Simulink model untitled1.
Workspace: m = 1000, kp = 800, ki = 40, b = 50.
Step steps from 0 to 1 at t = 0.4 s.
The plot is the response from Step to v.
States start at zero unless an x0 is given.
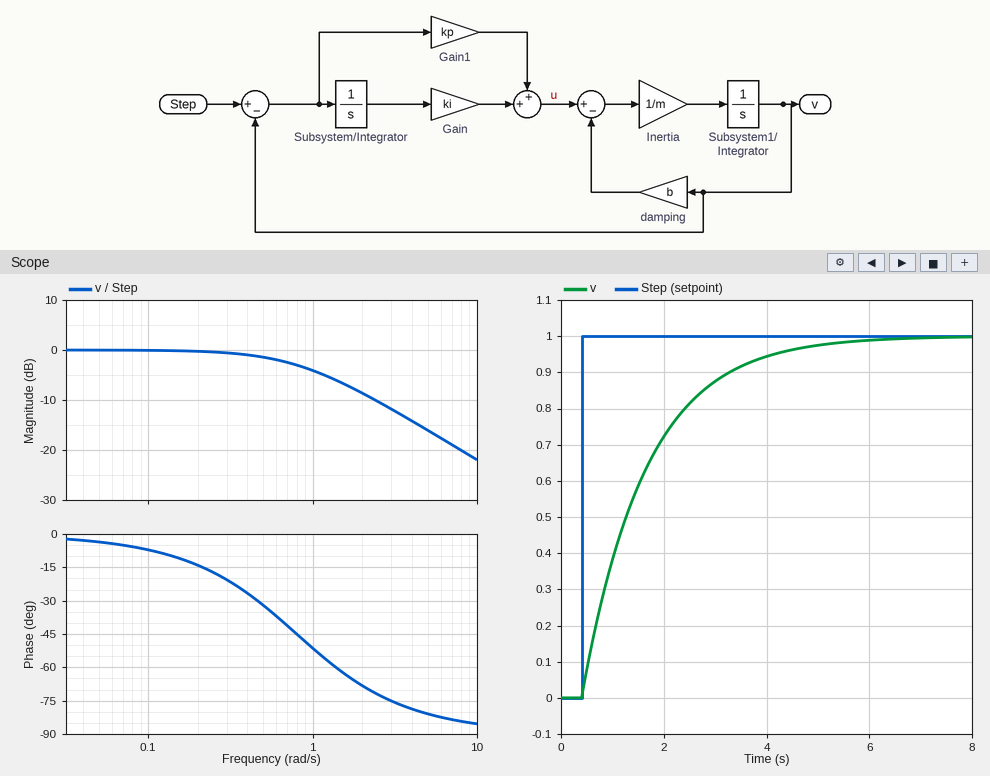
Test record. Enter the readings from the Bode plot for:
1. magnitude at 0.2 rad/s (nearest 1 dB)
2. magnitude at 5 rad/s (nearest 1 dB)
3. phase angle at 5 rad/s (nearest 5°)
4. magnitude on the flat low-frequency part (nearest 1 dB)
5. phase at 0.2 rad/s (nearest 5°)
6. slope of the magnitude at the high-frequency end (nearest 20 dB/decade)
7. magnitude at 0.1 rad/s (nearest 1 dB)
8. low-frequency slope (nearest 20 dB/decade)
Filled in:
0 dB
-16 dB
-80°
0 dB
-15°
-20 dB/decade
0 dB
0 dB/decade
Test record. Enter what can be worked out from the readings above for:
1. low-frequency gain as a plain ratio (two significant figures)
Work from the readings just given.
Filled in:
1.0
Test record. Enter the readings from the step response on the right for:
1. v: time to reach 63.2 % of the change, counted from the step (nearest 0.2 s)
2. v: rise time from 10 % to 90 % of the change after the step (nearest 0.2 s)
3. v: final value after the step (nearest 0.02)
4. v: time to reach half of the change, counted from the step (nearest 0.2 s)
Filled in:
1.2 s
2.8 s
1.00
0.8 s
